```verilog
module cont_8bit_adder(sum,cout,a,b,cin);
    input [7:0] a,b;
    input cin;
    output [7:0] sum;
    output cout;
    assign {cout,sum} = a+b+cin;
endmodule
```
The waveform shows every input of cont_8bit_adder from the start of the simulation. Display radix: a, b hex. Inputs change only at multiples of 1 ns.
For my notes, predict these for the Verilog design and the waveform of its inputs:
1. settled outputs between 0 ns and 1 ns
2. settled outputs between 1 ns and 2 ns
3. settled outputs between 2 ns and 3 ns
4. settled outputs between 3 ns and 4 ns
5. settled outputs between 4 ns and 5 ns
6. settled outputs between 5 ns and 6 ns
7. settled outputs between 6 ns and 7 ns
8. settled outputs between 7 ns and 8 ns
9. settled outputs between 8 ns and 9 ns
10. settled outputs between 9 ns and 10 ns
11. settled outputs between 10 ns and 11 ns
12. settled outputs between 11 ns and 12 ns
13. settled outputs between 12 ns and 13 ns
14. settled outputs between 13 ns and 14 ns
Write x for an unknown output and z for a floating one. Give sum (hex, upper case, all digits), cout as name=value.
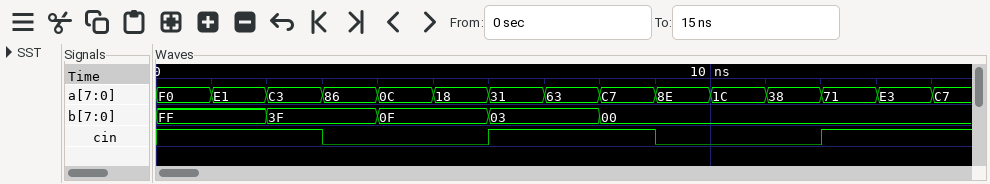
sum=F0, cout=1
sum=E1, cout=1
sum=03, cout=1
sum=C5, cout=0
sum=1B, cout=0
sum=27, cout=0
sum=35, cout=0
sum=67, cout=0
sum=C8, cout=0
sum=8E, cout=0
sum=1C, cout=0
sum=38, cout=0
sum=72, cout=0
sum=E4, cout=0
